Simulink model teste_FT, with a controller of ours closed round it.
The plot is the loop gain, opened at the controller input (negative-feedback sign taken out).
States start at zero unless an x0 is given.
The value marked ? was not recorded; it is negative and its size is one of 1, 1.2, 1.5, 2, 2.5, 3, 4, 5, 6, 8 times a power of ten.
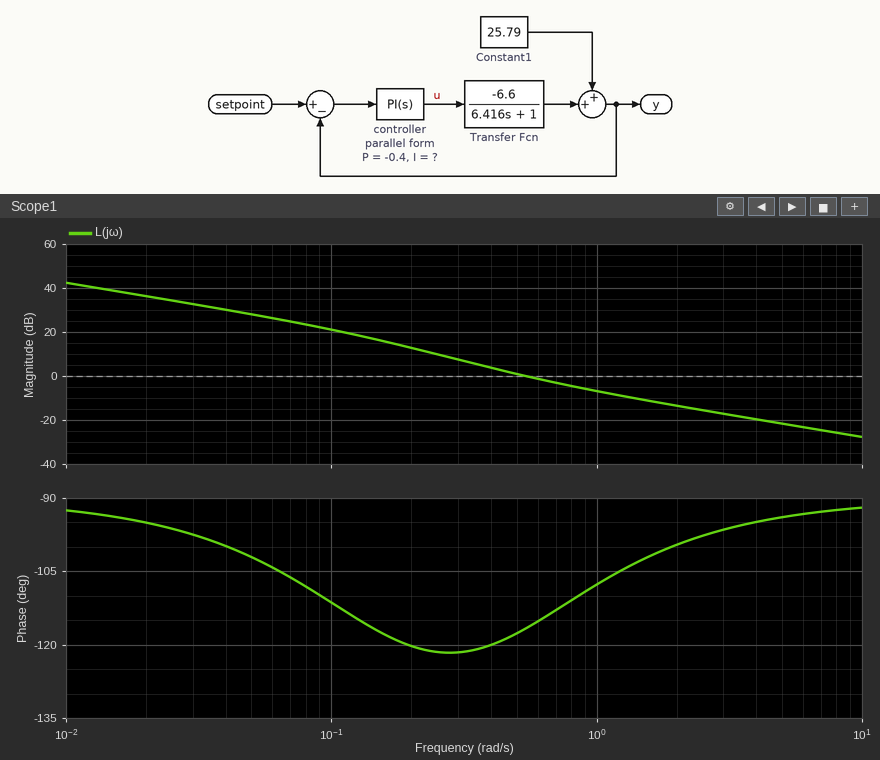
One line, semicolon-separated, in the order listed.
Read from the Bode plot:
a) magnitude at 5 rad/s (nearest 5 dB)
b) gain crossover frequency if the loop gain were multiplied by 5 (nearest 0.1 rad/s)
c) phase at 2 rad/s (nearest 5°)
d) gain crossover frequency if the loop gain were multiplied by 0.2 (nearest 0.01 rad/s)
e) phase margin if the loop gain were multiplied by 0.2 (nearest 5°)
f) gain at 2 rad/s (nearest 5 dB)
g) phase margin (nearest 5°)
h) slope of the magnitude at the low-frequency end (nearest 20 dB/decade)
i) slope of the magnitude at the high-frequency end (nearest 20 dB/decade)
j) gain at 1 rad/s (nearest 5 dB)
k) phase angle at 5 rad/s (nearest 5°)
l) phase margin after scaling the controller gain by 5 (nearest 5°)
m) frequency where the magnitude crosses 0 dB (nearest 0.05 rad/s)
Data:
-20 dB; 2.1 rad/s; -100°; 0.18 rad/s; 60°; -15 dB; 65°; -20 dB/decade; -20 dB/decade; -5 dB; -95°; 80°; 0.55 rad/s
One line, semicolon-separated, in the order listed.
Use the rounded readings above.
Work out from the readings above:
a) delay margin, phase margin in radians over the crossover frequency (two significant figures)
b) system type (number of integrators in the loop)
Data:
2.1 s; 1
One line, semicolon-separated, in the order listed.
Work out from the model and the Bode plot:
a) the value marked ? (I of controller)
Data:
-0.2
